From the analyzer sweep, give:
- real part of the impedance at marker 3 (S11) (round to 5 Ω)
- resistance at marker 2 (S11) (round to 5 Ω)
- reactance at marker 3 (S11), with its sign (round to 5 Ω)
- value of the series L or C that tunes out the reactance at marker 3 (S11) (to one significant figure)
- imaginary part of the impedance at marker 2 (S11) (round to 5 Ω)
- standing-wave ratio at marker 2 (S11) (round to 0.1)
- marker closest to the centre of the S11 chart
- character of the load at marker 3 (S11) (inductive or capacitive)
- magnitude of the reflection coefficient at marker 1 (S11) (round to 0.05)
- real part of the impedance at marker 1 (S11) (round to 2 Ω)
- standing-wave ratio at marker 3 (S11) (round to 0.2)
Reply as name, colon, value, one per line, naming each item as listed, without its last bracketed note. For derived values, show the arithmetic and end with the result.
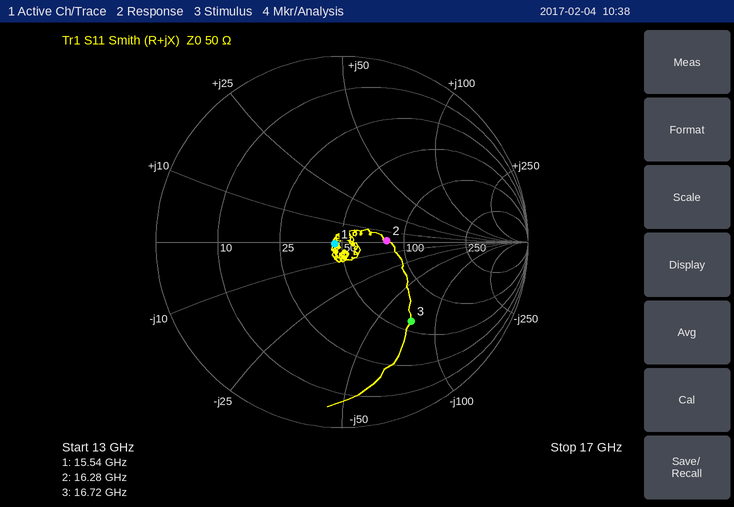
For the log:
real part of the impedance at marker 3 (S11): 60 Ω
resistance at marker 2 (S11): 80 Ω
reactance at marker 3 (S11), with its sign: -75 Ω
value of the series L or C that tunes out the reactance at marker 3 (S11): L = 75 Ω/(2π × 16.72 GHz) ≈ 714 pH, so 700 pH to one significant figure
imaginary part of the impedance at marker 2 (S11): 0 Ω
standing-wave ratio at marker 2 (S11): 1.6
marker closest to the centre of the S11 chart: marker 1
character of the load at marker 3 (S11): capacitive
magnitude of the reflection coefficient at marker 1 (S11): 0.05
real part of the impedance at marker 1 (S11): 46 Ω
standing-wave ratio at marker 3 (S11): 3.6
